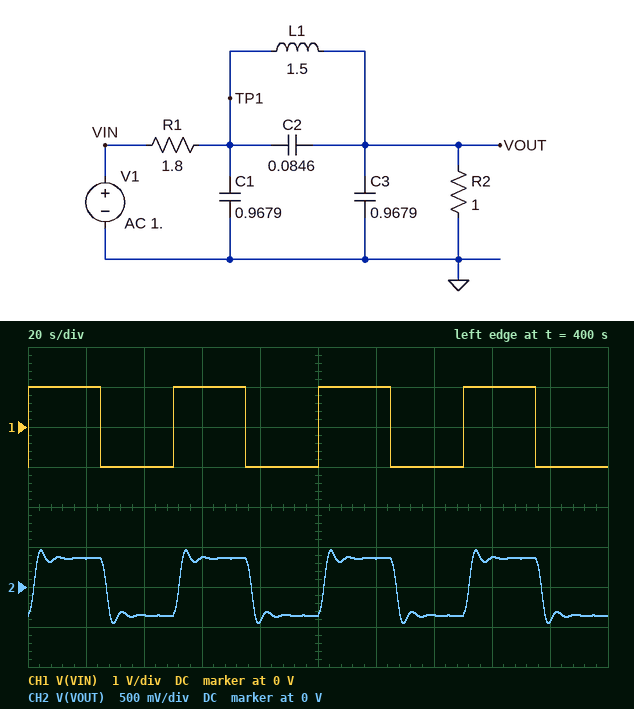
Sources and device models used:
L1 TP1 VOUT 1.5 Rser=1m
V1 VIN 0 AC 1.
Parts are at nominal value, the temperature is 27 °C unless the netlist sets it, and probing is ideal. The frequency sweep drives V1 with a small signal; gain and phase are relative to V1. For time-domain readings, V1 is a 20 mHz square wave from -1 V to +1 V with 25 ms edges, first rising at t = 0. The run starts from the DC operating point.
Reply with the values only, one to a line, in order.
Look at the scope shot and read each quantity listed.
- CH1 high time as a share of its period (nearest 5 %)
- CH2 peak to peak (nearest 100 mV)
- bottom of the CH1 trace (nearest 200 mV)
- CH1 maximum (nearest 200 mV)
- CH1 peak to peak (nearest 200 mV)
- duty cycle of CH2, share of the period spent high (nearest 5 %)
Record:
50 %
900 mV
-1.0 V
1.0 V
2.0 V
50 %
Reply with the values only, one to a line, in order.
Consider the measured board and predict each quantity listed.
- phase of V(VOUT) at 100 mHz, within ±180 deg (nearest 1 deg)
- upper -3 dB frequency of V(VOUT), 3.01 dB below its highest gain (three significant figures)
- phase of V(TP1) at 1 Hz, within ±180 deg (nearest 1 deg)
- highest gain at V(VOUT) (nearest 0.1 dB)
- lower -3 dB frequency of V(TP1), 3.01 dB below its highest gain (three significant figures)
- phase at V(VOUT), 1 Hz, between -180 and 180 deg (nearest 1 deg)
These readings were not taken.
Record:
-66 deg
181 mHz
-85 deg
-8.6 dB
119 mHz
-76 deg
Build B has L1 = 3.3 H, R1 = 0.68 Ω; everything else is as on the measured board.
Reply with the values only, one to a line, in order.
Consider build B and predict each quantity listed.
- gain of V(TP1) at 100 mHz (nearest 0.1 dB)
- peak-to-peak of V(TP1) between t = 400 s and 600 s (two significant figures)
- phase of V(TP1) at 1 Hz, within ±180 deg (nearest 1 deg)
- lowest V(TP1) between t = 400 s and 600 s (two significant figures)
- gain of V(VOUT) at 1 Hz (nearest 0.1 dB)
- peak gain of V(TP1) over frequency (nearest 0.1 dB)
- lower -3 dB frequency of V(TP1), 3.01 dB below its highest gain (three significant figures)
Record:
-1.0 dB
2.1 V
-77 deg
-1.0 V
-35.9 dB
-0.8 dB
35.7 mHz
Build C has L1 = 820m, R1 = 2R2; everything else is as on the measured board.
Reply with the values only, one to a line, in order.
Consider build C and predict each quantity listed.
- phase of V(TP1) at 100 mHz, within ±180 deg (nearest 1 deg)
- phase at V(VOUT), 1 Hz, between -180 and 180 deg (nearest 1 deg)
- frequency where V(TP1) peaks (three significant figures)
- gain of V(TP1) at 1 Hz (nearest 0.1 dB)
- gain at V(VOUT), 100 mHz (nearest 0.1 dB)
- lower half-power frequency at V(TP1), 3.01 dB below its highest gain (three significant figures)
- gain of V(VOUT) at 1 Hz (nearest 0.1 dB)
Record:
-14 deg
-77 deg
233 mHz
-23.0 dB
-10.9 dB
187 mHz
-48.7 dB
